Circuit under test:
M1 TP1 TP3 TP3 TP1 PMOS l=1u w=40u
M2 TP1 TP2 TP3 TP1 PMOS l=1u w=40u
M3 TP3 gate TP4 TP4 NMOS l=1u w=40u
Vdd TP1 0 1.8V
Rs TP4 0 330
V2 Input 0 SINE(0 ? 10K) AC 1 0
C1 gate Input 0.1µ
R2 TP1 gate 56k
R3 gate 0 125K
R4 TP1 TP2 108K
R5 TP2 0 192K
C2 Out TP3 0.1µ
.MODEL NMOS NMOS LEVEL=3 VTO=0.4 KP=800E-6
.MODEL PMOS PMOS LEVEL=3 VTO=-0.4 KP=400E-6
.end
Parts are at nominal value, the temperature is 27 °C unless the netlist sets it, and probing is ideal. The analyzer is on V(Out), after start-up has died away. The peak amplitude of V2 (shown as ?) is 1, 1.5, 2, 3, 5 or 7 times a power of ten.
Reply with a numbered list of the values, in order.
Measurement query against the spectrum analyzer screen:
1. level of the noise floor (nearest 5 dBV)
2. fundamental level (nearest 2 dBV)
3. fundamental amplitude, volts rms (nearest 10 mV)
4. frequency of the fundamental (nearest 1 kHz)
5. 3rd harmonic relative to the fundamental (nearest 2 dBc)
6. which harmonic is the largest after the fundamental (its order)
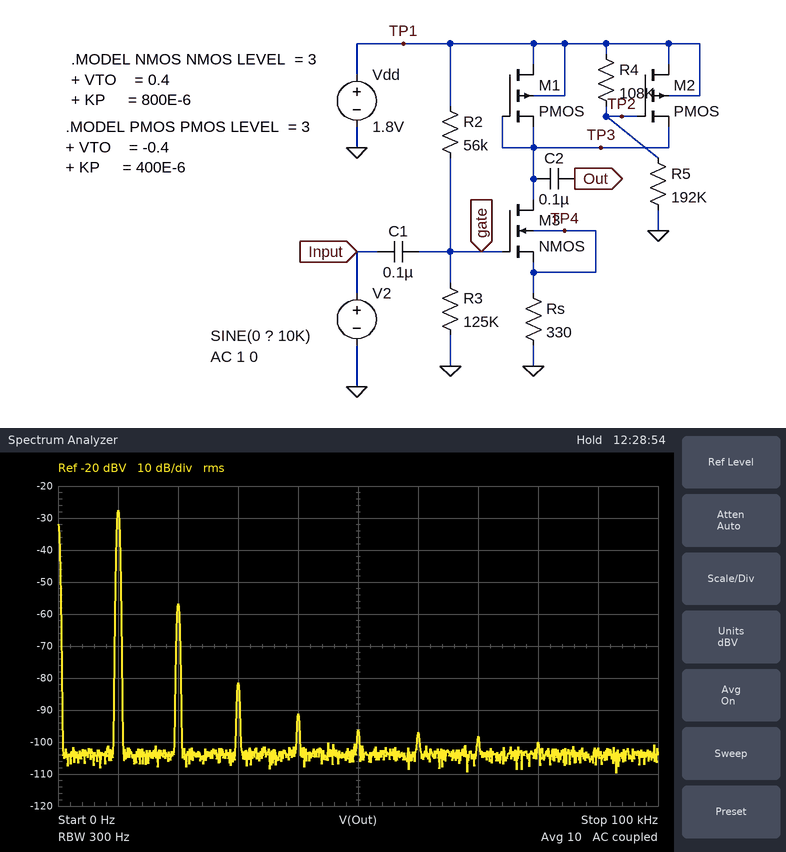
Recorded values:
1. -105 dBV
2. -28 dBV
3. 40 mV
4. 10 kHz
5. -54 dBc
6. 2
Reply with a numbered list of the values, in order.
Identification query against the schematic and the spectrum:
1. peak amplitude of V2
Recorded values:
1. 150 mV
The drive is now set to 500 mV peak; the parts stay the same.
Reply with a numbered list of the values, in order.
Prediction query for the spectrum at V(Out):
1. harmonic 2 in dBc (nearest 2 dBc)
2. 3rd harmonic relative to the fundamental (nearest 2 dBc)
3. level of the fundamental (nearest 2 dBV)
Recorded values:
1. -12 dBc
2. -28 dBc
3. -16 dBV
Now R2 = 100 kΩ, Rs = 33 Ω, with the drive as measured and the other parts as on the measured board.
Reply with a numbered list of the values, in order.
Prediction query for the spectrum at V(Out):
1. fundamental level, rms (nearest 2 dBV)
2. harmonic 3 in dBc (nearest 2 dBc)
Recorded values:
1. -20 dBV
2. -40 dBc
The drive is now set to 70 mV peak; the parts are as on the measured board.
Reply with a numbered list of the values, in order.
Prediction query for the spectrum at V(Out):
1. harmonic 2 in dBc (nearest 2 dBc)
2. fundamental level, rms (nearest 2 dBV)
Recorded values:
1. -36 dBc
2. -34 dBV
